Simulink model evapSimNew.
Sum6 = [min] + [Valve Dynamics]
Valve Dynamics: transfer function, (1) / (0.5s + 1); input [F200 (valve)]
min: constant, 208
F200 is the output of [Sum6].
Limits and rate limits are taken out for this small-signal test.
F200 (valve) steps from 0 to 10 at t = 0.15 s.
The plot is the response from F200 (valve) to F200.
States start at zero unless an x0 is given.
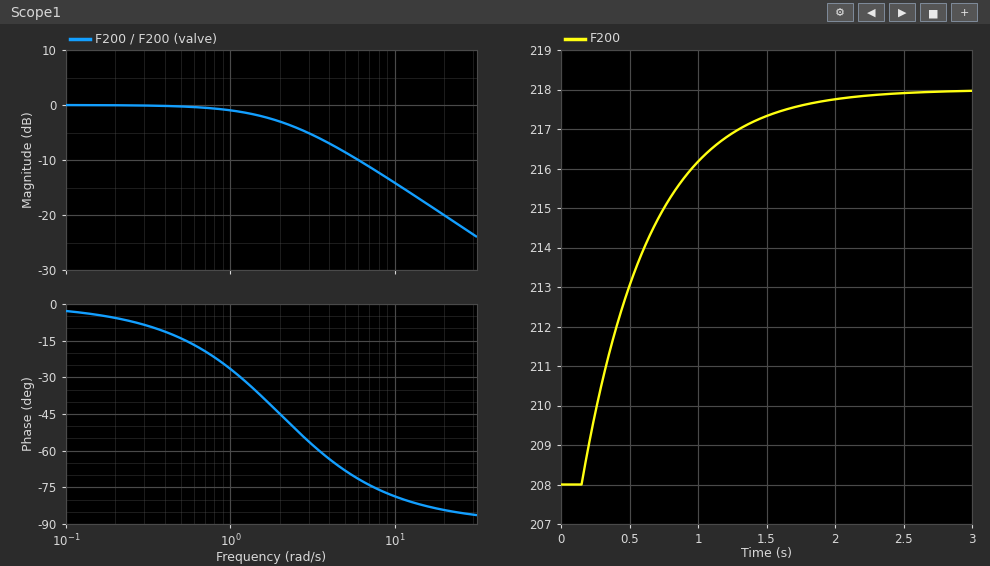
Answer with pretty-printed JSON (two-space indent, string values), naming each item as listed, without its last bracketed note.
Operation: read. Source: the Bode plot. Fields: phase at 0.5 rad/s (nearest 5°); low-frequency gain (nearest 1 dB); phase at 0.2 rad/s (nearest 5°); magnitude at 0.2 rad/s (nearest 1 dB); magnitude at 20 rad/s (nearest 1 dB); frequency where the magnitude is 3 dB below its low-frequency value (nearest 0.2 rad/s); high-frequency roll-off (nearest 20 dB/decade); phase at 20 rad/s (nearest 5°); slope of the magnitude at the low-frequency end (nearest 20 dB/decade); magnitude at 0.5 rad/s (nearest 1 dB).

{
  "phase at 0.5 rad/s": "-15°",
  "low-frequency gain": "0 dB",
  "phase at 0.2 rad/s": "-5°",
  "magnitude at 0.2 rad/s": "0 dB",
  "magnitude at 20 rad/s": "-20 dB",
  "frequency where the magnitude is 3 dB below its low-frequency value": "2.0 rad/s",
  "high-frequency roll-off": "-20 dB/decade",
  "phase at 20 rad/s": "-85°",
  "slope of the magnitude at the low-frequency end": "0 dB/decade",
  "magnitude at 0.5 rad/s": "0 dB"
}
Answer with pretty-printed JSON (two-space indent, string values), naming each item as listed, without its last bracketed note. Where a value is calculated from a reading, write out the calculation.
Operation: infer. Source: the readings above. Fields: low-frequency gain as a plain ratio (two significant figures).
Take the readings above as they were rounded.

{
  "low-frequency gain as a plain ratio": "10^(0 / 20) = 1.0"
}
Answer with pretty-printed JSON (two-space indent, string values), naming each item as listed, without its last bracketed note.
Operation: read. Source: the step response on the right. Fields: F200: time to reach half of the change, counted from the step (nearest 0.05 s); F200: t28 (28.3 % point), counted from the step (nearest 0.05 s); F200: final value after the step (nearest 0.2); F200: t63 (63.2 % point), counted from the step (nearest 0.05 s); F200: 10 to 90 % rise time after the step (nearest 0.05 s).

{
  "F200: time to reach half of the change, counted from the step": "0.35 s",
  "F200: t28 (28.3 % point), counted from the step": "0.15 s",
  "F200: final value after the step": "218.0",
  "F200: t63 (63.2 % point), counted from the step": "0.50 s",
  "F200: 10 to 90 % rise time after the step": "1.10 s"
}
